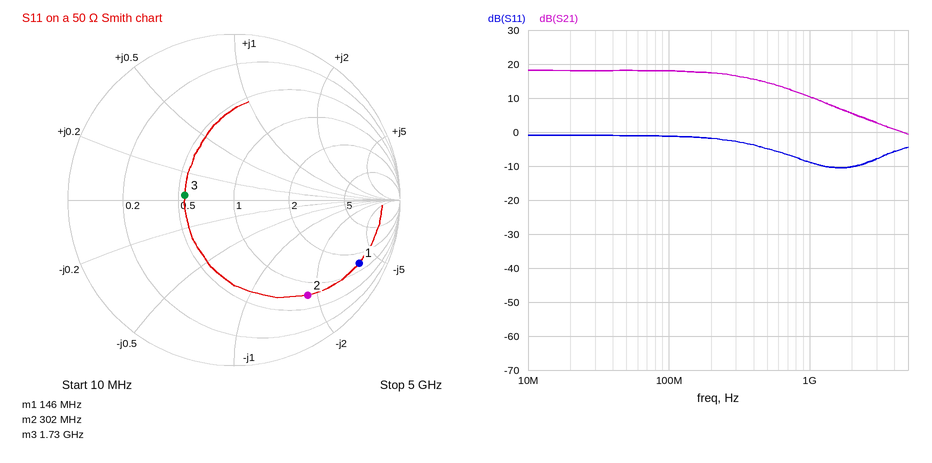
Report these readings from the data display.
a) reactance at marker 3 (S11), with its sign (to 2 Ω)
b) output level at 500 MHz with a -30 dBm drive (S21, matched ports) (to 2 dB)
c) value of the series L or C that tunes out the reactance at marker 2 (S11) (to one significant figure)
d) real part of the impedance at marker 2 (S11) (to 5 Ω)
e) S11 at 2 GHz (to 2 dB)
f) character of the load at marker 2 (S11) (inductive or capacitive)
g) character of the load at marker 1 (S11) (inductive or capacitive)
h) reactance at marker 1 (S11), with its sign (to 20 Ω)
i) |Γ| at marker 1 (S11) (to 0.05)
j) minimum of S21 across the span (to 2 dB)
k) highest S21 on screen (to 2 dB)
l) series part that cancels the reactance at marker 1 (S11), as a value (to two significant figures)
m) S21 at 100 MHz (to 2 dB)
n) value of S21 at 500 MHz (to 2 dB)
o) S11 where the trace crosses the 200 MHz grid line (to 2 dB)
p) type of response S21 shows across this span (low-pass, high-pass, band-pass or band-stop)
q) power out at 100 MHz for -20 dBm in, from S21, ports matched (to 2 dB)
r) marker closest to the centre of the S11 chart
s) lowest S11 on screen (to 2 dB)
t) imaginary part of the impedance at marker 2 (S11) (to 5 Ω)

+2 Ω
-16 dBm
50 nH
35 Ω
-10 dB
capacitive
capacitive
-180 Ω
0.85
0 dB
18 dB
200 nH
18 dB
14 dB
-2 dB
low-pass
-2 dBm
marker 3
-10 dB
-90 Ω
